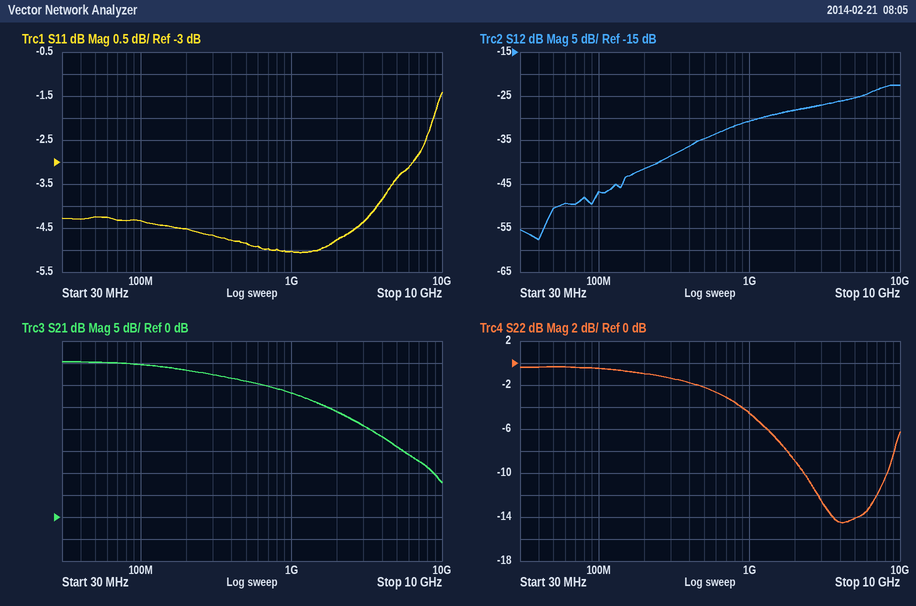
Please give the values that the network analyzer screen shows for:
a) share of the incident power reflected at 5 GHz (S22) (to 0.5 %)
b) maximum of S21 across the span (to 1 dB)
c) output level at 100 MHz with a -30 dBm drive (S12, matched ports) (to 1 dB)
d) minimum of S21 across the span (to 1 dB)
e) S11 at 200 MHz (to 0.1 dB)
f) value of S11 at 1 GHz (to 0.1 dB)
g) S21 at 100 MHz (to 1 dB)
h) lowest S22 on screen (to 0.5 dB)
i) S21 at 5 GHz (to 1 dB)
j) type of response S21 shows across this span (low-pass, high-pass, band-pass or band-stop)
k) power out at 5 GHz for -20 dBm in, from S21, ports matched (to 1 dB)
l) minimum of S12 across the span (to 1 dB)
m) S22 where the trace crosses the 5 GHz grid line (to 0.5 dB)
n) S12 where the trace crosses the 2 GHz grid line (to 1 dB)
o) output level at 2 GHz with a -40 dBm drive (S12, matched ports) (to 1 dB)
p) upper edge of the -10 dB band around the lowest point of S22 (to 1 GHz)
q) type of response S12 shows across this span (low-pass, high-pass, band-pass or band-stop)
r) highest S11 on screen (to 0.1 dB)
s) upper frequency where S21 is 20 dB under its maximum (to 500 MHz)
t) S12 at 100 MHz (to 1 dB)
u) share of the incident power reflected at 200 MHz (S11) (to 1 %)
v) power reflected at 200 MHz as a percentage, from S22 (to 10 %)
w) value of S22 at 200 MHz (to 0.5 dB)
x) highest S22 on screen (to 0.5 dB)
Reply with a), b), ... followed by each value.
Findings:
a) 4.0 %
b) 35 dB
c) -77 dBm
d) 8 dB
e) -4.5 dB
f) -5.0 dB
g) 35 dB
h) -14.5 dB
i) 16 dB
j) low-pass
k) -4 dBm
l) -58 dB
m) -14.0 dB
n) -28 dB
o) -68 dBm
p) 8 GHz
q) high-pass
r) -1.4 dB
s) 5.5 GHz
t) -47 dB
u) 35 %
v) 80 %
w) -1.0 dB
x) -0.5 dB
